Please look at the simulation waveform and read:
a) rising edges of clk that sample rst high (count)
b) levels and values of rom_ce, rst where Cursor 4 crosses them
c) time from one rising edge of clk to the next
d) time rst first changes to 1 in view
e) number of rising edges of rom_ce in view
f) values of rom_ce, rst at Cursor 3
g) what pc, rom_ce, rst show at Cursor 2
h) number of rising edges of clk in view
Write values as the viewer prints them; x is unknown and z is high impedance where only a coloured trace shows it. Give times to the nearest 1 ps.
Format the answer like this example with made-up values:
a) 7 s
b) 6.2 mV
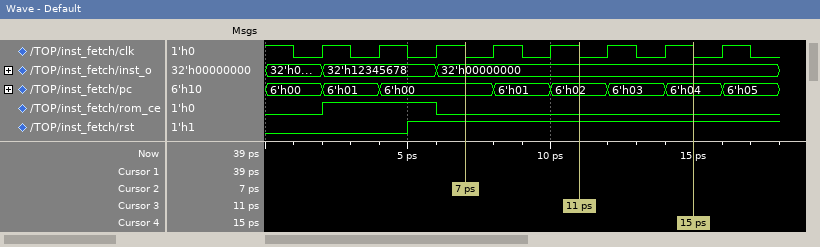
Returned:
a) 6
b) rom_ce=0, rst=1
c) 2 ps
d) 5 ps
e) 1
f) rom_ce=0, rst=1
g) pc=6'h00, rom_ce=0, rst=1
h) 8
